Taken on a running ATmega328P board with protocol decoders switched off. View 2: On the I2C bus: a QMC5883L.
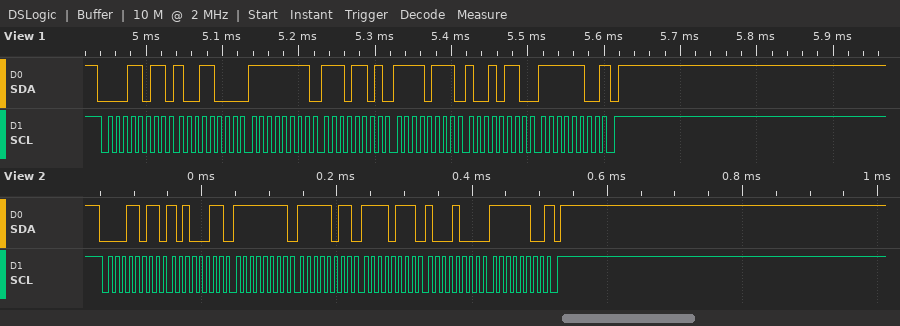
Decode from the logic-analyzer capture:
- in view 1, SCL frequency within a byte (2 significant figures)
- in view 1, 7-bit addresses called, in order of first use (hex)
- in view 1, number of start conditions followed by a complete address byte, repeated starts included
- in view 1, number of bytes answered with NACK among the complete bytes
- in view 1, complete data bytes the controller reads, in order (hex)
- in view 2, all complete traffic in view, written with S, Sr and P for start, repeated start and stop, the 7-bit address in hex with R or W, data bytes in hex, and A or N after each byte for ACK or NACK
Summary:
100 kHz
0x0D
1
1
98 FF ED F7 96 FC
S 0DR A A3 A FF A FB A F7 A 88 A FC N P
